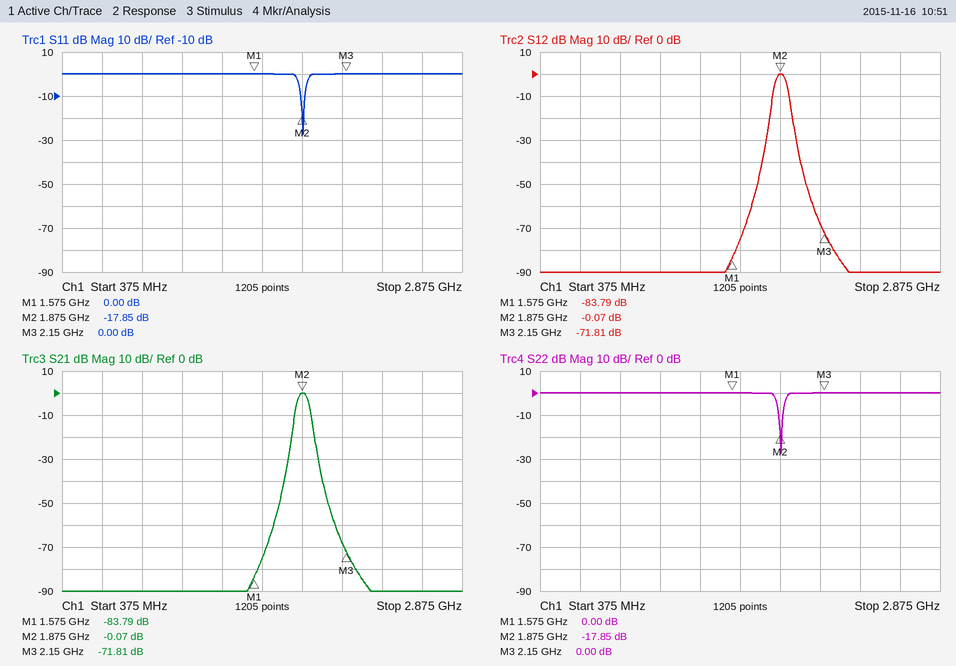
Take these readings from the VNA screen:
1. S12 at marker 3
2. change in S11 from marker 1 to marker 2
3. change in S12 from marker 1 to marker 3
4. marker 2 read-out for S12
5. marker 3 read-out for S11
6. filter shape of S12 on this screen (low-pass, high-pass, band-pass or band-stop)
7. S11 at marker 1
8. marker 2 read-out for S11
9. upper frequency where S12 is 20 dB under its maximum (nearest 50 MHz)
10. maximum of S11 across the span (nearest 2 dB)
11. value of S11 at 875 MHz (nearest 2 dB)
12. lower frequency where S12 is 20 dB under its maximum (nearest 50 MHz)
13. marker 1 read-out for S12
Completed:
-71.81 dB
-17.85 dB
11.98 dB
-0.07 dB
0.00 dB
band-pass
0.00 dB
-17.85 dB
1.95 GHz
0 dB
0 dB
1.80 GHz
-83.79 dB
